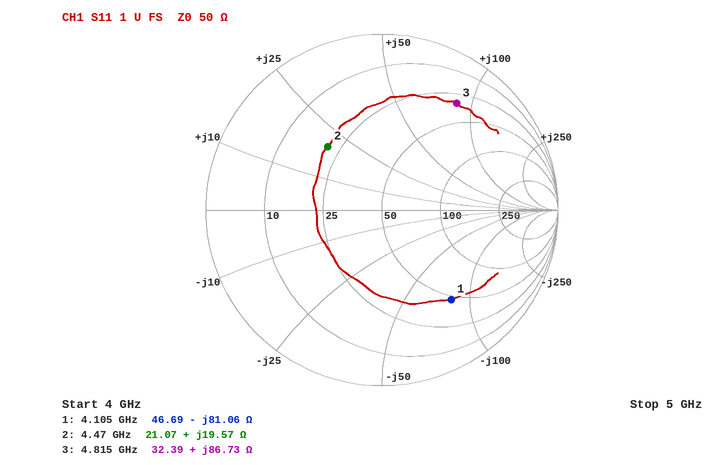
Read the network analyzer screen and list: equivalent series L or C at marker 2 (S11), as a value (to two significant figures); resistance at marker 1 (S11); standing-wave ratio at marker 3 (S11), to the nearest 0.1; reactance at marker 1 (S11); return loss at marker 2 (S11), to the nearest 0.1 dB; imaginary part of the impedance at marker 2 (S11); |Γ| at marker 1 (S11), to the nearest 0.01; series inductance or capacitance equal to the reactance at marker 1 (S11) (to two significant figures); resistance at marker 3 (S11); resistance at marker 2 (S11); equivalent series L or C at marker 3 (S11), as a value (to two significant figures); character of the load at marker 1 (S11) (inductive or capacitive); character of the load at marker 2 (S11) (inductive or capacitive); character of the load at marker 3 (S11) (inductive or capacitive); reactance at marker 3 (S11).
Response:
700 pH
46.69 Ω
6.7
-81.06 Ω
6.5 dB
+19.57 Ω
0.64
480 fF
32.39 Ω
21.07 Ω
2.9 nH
capacitive
inductive
inductive
+86.73 Ω
